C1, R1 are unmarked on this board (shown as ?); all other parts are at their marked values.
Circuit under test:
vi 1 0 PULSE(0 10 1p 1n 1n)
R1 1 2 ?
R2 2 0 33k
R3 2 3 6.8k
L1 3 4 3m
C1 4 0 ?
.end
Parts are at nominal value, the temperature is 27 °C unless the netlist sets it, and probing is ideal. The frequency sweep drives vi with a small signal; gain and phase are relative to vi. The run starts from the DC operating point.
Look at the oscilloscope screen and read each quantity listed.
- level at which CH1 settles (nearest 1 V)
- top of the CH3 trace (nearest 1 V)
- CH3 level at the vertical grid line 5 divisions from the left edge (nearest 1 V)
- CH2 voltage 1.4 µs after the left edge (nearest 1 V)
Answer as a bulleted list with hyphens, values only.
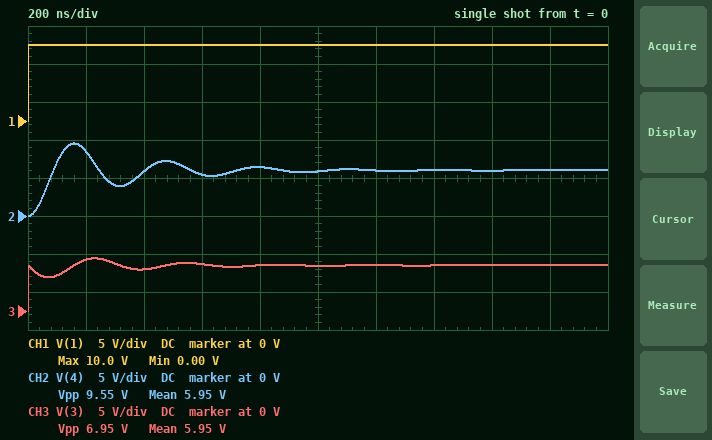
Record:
- 10 V
- 7 V
- 6 V
- 6 V
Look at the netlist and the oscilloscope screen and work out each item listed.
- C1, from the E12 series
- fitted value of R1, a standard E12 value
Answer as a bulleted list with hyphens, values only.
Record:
- 820 fF
- 22 kΩ
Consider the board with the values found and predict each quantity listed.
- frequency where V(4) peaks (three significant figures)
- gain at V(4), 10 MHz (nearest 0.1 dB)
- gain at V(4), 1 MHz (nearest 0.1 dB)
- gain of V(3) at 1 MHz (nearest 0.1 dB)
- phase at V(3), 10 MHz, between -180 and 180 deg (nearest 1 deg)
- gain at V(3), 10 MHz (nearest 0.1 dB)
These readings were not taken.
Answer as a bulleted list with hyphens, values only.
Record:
- 3.12 MHz
- -23.3 dB
- -3.6 dB
- -4.5 dB
- 7 deg
- -4.5 dB
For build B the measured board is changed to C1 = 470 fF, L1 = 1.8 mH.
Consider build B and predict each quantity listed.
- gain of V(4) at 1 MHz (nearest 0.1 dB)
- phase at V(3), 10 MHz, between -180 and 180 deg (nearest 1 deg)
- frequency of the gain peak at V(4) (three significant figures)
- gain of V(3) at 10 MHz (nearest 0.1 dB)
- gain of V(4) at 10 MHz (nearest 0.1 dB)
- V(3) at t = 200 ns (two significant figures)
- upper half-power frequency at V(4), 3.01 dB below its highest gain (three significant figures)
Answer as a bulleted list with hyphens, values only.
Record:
- -4.2 dB
- 14 deg
- 5.33 MHz
- -4.7 dB
- -12.1 dB
- 5.7 V
- 6.16 MHz
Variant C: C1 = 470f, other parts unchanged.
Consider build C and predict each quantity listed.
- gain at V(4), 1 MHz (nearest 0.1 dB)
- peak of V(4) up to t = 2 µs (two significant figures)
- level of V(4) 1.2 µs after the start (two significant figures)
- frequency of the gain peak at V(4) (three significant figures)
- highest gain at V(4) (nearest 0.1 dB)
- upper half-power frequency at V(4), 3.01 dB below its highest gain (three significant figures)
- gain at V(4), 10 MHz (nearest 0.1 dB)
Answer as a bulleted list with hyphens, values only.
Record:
- -4.0 dB
- 10 V
- 5.9 V
- 4.17 MHz
- 7.7 dB
- 4.68 MHz
- -17.7 dB
